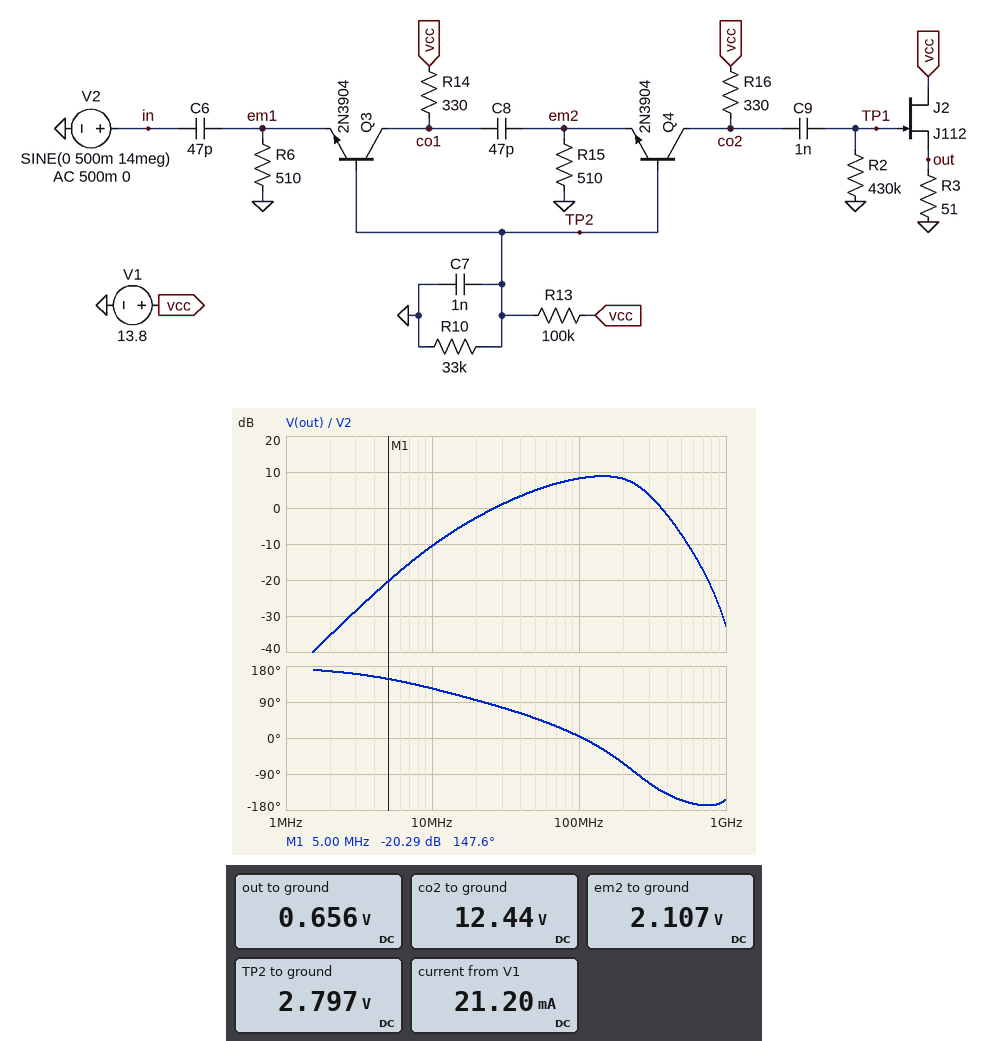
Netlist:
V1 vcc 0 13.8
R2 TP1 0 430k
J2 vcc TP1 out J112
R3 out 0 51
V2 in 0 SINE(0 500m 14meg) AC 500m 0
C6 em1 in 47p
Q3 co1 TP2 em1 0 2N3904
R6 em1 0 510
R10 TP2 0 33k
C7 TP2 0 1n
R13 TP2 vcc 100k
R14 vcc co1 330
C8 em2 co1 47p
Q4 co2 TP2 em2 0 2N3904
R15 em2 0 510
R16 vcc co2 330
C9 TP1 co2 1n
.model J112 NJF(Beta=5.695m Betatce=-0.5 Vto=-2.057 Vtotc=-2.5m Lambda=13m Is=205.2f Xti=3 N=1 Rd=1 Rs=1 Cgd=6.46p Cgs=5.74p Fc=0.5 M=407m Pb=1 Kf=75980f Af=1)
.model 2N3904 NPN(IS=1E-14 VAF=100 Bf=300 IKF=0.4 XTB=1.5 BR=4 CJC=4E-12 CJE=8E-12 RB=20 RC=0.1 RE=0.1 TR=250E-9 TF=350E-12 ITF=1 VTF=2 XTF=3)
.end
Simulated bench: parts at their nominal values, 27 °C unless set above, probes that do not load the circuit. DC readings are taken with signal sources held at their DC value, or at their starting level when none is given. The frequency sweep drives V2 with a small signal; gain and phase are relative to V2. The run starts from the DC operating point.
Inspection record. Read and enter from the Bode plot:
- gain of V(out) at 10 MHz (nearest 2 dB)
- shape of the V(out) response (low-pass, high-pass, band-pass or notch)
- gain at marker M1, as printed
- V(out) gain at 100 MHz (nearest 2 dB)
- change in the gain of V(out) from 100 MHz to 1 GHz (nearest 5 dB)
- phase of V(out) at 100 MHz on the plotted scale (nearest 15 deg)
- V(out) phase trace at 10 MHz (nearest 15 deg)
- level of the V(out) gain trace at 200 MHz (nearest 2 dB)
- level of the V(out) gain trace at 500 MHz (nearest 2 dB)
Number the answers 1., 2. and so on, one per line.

1. -10 dB
2. band-pass
3. -20.29 dB
4. 8 dB
5. -40 dB
6. 0 deg
7. 120 deg
8. 8 dB
9. -8 dB
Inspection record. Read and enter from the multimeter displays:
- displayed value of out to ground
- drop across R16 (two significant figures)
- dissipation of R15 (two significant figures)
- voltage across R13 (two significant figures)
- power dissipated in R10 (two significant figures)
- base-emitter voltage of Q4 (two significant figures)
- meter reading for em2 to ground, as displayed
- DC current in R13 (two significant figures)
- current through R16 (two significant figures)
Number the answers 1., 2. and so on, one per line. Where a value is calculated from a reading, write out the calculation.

1. 0.656 V
2. 13.8 V - 12.44 V = 1.4 V
3. (2.107 V)^2 / 510 Ω = 8.7 mW
4. 13.8 V - 2.797 V = 11 V
5. (2.797 V)^2 / 33 kΩ = 240 µW
6. 2.797 V - 2.107 V = 690 mV
7. 2.107 V
8. (13.8 V - 2.797 V) / 100 kΩ = 110 µA
9. (13.8 V - 12.44 V) / 330 Ω = 4.1 mA
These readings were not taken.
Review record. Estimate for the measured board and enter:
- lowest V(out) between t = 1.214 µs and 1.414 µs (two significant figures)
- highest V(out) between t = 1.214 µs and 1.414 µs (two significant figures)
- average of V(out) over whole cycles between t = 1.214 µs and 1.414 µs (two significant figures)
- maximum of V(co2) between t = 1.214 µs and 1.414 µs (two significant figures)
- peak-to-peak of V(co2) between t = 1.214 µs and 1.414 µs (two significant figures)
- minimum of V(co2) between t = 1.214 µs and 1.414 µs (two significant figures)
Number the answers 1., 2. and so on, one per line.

1. 430 mV
2. 900 mV
3. 660 mV
4. 13 V
5. 1.0 V
6. 12 V
